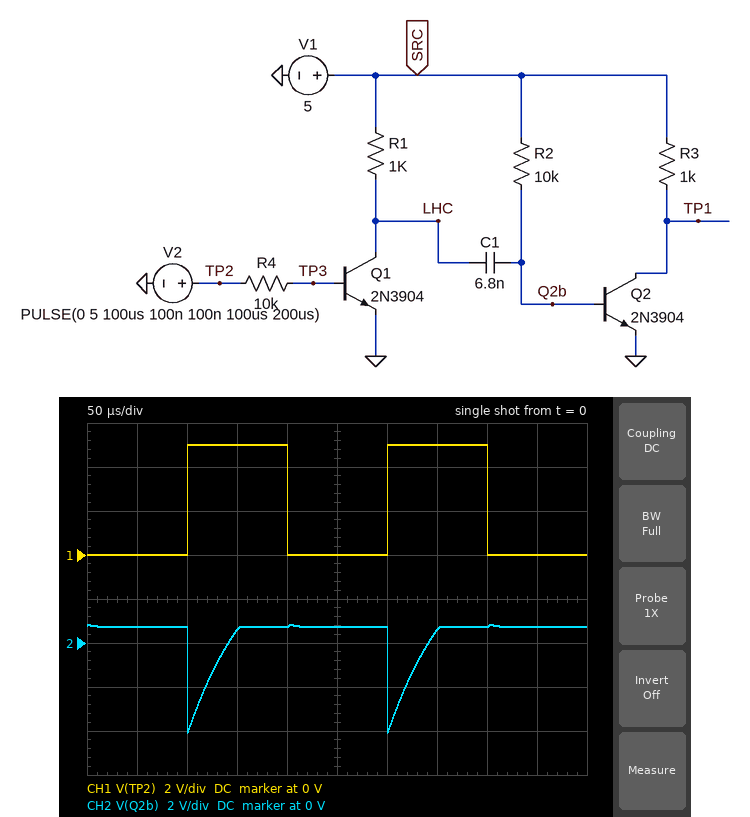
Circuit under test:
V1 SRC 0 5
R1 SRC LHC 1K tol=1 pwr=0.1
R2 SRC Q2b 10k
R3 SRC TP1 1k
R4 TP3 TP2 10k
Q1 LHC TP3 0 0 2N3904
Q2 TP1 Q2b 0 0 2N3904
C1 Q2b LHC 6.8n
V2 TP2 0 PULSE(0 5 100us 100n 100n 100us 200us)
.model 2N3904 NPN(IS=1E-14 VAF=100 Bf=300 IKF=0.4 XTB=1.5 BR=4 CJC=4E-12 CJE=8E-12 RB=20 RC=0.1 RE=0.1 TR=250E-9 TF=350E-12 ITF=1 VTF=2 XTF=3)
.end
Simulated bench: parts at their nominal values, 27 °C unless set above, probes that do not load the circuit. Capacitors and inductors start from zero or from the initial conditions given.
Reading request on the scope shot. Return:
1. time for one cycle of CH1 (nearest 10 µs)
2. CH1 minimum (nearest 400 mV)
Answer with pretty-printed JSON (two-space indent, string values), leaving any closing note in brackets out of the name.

{
  "time for one cycle of CH1": "200 µs",
  "CH1 minimum": "0 V"
}
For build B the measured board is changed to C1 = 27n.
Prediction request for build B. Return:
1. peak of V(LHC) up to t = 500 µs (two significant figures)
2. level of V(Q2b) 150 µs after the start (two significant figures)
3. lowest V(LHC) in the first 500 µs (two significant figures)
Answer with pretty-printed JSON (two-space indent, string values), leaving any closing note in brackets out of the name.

{
  "peak of V(LHC) up to t = 500 µs": "4.9 V",
  "level of V(Q2b) 150 µs after the start": "-2.6 V",
  "lowest V(LHC) in the first 500 µs": "41 mV"
}
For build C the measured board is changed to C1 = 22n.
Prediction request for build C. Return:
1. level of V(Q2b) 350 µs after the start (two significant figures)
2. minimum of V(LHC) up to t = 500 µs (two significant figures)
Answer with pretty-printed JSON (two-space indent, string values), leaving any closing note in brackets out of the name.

{
  "level of V(Q2b) 350 µs after the start": "-2.3 V",
  "minimum of V(LHC) up to t = 500 µs": "41 mV"
}
